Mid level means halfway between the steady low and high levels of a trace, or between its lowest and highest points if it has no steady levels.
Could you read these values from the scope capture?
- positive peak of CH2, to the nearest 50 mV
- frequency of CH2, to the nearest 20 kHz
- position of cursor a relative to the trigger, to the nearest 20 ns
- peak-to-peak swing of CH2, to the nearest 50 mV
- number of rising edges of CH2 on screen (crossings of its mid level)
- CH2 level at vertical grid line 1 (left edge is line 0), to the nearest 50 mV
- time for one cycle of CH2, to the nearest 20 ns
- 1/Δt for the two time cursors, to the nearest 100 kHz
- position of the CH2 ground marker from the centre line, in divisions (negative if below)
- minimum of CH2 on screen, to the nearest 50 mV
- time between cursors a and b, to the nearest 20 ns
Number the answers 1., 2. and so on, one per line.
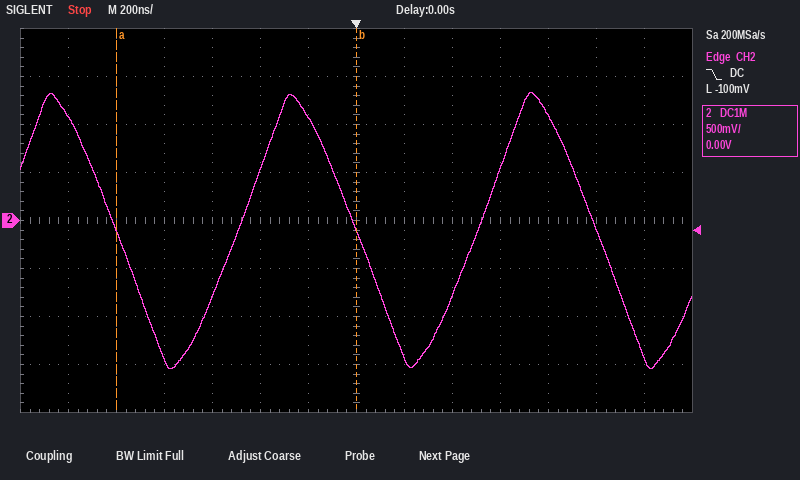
1. 1.35 V
2. 1.00 MHz
3. -1.00 µs
4. 2.90 V
5. 2
6. 1.10 V
7. 1.00 µs
8. 1.0 MHz
9. 0.0 div
10. -1.55 V
11. 1.00 µs
